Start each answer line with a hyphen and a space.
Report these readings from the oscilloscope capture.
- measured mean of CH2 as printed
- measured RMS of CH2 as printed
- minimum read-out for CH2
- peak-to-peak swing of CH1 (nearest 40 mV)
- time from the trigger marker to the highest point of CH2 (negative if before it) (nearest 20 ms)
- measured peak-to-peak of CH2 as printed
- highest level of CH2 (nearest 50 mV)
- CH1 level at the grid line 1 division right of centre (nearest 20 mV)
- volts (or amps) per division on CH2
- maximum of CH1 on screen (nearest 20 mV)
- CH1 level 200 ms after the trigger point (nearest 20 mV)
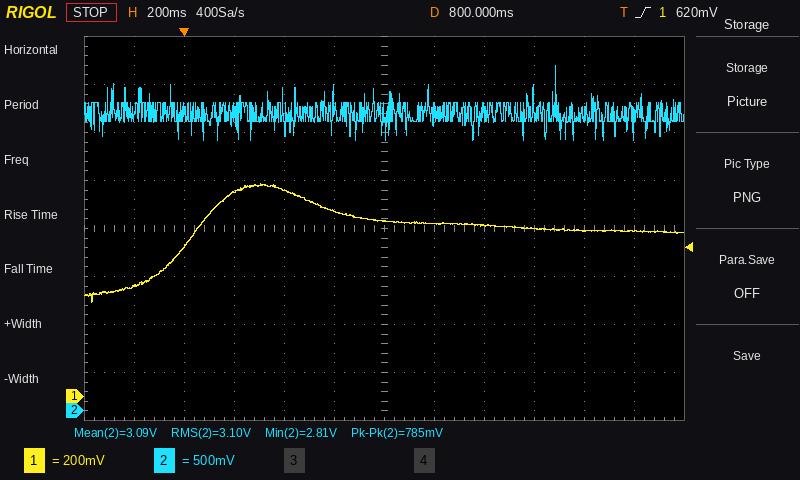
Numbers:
- 3.09 V
- 3.10 V
- 2.81 V
- 480 mV
- +1.48 s
- 785 mV
- 3.60 V
- 720 mV
- 500 mV
- 880 mV
- 860 mV
